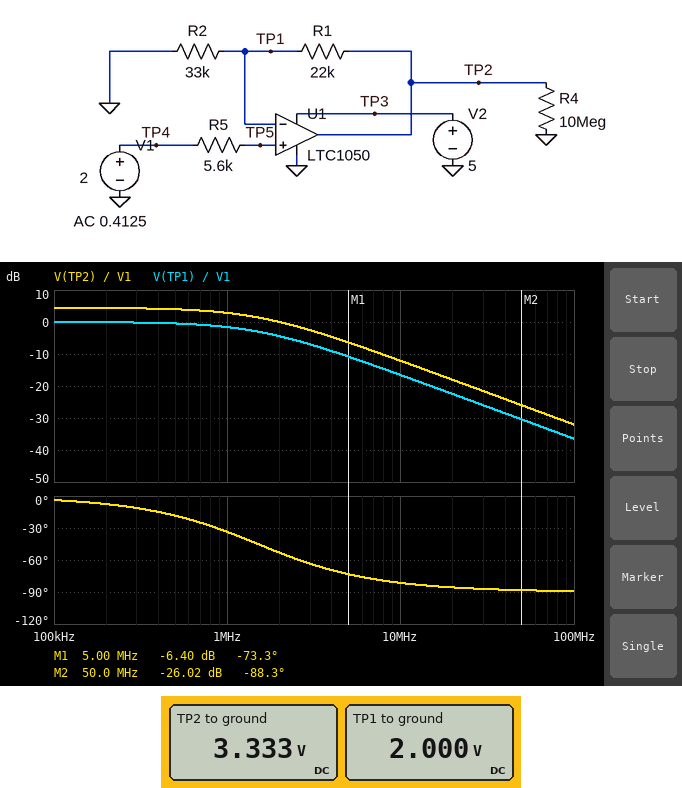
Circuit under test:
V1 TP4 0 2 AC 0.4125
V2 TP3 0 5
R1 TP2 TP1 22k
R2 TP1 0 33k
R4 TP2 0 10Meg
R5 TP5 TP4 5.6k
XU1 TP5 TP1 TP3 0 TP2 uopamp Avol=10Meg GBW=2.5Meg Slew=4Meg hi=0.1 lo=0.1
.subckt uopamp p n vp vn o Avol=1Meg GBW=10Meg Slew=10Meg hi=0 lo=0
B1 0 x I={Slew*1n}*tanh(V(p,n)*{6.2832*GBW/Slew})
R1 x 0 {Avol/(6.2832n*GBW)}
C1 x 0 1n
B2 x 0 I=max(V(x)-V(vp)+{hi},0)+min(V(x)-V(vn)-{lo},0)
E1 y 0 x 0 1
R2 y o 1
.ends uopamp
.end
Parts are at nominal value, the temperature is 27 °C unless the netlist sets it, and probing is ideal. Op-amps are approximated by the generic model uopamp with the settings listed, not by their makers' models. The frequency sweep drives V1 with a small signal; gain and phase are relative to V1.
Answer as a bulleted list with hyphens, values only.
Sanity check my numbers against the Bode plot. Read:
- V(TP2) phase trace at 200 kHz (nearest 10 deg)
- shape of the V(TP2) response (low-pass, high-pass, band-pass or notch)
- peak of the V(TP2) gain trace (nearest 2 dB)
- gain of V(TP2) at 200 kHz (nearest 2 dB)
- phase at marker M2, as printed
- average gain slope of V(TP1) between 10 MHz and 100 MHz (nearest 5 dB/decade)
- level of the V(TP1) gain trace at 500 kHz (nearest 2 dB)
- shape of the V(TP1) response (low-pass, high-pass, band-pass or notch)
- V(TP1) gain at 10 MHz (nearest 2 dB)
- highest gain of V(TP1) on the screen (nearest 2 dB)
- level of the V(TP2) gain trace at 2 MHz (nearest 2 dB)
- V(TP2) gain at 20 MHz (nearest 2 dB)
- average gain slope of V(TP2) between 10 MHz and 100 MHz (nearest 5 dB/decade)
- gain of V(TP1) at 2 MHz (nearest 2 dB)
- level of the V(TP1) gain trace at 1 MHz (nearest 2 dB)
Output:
- -10 deg
- low-pass
- 4 dB
- 4 dB
- -88.3 deg
- -20 dB/decade
- 0 dB
- low-pass
- -16 dB
- 0 dB
- 0 dB
- -18 dB
- -20 dB/decade
- -4 dB
- -2 dB
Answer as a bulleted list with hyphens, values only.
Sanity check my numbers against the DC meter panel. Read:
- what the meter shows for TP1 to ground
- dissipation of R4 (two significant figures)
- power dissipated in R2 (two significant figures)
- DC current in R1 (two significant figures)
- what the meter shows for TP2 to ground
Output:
- 2.000 V
- 1.1 µW
- 120 µW
- 61 µA
- 3.333 V
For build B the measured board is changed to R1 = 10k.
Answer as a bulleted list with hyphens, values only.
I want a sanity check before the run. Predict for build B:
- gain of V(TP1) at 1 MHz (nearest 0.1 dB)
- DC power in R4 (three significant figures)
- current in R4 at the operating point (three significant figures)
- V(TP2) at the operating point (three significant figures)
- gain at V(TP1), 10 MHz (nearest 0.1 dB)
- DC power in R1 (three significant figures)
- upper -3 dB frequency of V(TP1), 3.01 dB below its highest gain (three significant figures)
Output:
- -1.0 dB
- 679 nW
- 261 nA
- 2.61 V
- -14.5 dB
- 36.7 µW
- 1.92 MHz
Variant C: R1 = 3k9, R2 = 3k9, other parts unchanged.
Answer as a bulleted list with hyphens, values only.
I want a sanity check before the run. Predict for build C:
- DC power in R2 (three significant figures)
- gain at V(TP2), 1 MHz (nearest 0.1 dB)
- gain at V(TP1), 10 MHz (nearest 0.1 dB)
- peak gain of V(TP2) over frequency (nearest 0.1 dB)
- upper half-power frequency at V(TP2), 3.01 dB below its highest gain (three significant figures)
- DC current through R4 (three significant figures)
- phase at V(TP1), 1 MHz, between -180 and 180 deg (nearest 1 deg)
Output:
- 1.03 mW
- 3.9 dB
- -18.1 dB
- 6.0 dB
- 1.25 MHz
- 400 nA
- -39 deg
